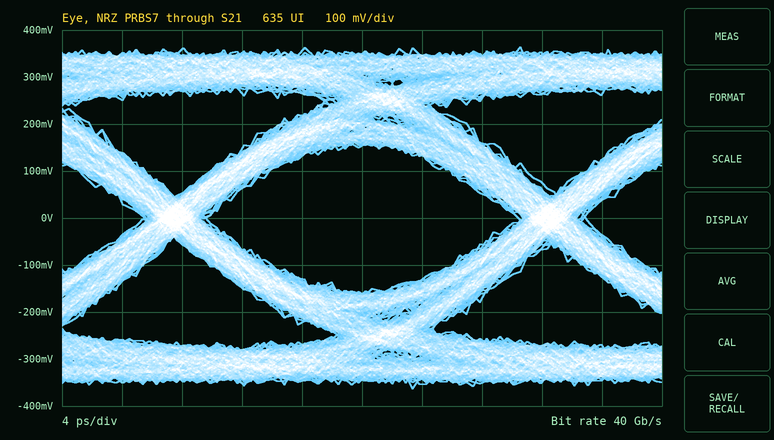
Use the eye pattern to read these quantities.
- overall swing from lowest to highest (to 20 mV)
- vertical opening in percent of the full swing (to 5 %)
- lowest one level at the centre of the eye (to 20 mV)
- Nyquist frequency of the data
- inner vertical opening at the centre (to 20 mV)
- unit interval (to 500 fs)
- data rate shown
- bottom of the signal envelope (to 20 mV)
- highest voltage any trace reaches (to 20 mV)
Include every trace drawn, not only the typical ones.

720 mV
45 %
160 mV
20 GHz
320 mV
25.0 ps
40 Gb/s
-360 mV
360 mV
